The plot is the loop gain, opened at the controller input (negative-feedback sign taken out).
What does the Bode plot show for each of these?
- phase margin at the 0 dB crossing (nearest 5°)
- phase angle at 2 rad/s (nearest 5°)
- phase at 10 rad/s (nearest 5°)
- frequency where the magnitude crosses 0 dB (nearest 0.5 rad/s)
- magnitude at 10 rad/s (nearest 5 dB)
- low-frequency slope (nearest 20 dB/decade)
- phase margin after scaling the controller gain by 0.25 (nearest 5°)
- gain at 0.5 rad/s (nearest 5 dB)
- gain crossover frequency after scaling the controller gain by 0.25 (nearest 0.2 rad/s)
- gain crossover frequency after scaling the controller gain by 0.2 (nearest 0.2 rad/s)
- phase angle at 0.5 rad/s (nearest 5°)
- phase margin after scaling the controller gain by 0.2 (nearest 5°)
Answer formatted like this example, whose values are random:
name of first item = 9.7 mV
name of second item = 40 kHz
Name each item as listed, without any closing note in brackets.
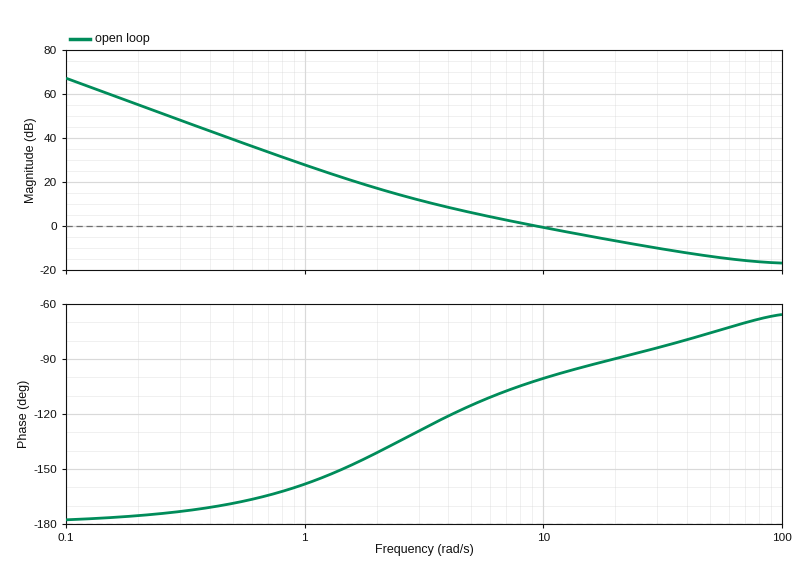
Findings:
phase margin at the 0 dB crossing = 80°
phase angle at 2 rad/s = -140°
phase at 10 rad/s = -100°
frequency where the magnitude crosses 0 dB = 9.5 rad/s
magnitude at 10 rad/s = 0 dB
low-frequency slope = -40 dB/decade
phase margin after scaling the controller gain by 0.25 = 50°
gain at 0.5 rad/s = 40 dB
gain crossover frequency after scaling the controller gain by 0.25 = 3.0 rad/s
gain crossover frequency after scaling the controller gain by 0.2 = 2.6 rad/s
phase angle at 0.5 rad/s = -170°
phase margin after scaling the controller gain by 0.2 = 45°
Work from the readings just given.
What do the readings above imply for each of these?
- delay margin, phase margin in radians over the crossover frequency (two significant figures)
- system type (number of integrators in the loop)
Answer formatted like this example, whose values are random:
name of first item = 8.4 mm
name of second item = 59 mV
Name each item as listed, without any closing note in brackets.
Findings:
delay margin, phase margin in radians over the crossover frequency = 0.15 s
system type = 2
